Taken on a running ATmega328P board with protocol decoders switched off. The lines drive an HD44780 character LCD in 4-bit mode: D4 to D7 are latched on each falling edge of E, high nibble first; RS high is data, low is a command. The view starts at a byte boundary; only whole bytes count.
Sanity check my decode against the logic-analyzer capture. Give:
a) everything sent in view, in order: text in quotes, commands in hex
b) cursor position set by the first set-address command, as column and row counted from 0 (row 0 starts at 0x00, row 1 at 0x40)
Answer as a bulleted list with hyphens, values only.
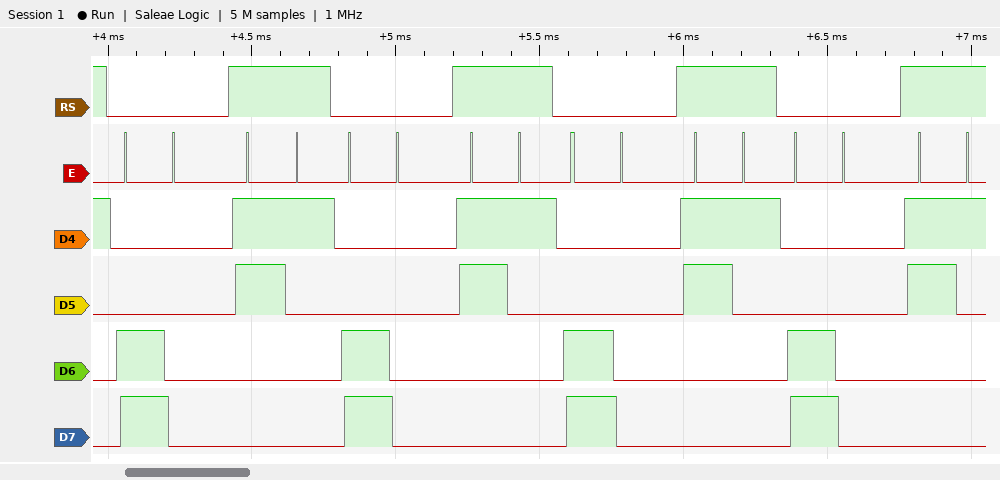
- 0xC0 "1" 0xC0 "1" 0xC0 "1" 0xC0 "1"
- column 0, row 1
